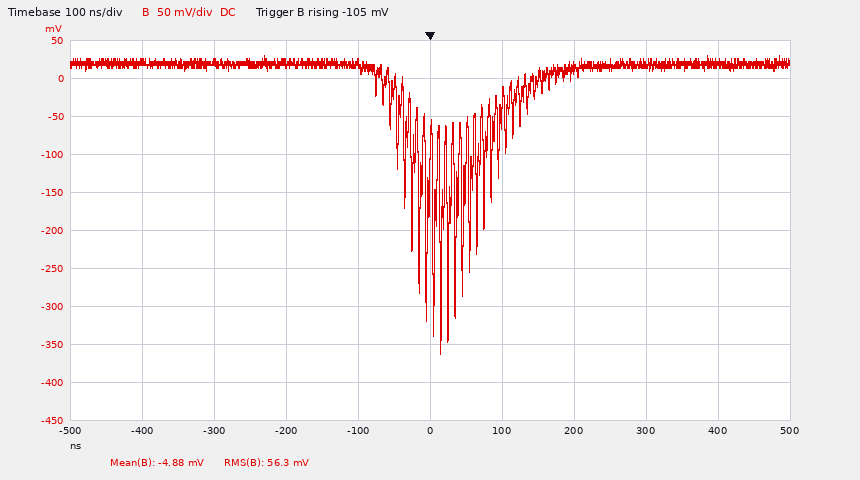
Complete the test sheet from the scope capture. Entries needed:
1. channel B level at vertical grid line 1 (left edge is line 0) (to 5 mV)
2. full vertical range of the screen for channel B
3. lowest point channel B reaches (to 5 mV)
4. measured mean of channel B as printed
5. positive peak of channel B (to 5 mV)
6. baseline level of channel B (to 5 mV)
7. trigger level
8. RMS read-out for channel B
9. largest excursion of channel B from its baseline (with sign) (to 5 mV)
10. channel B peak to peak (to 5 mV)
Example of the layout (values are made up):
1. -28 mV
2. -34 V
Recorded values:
1. 20 mV
2. 500 mV
3. -360 mV
4. -4.88 mV
5. 30 mV
6. 20 mV
7. -105 mV
8. 56.3 mV
9. -380 mV
10. 390 mV
